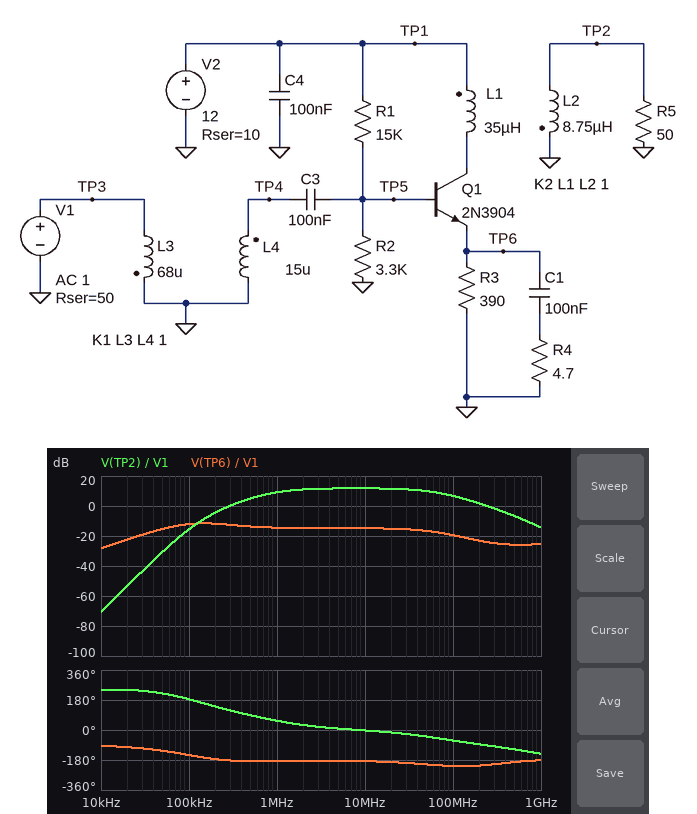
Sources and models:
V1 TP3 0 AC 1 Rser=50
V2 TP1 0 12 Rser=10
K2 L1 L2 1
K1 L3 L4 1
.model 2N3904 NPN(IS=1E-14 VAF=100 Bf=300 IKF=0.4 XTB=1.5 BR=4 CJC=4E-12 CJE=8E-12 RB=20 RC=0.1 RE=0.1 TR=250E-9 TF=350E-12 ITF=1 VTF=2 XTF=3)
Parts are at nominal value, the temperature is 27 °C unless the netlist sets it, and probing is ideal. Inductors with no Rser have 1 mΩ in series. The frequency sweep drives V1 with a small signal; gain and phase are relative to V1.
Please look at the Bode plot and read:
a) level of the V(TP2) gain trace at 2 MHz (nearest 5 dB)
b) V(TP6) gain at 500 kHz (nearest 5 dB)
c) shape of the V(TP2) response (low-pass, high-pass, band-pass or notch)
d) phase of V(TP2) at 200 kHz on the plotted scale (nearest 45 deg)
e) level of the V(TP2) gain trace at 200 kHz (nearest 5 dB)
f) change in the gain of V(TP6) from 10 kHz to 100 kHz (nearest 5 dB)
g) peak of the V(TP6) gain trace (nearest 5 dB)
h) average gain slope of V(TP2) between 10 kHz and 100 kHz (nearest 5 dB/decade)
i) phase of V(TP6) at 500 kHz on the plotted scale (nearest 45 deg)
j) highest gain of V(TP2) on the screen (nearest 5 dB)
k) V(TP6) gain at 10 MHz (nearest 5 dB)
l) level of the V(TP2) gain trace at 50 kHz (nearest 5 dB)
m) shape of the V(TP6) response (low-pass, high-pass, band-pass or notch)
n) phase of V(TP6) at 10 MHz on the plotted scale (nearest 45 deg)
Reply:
10 dB
-15 dB
band-pass
135 deg
-5 dB
15 dB
-10 dB
55 dB/decade
-180 deg
10 dB
-15 dB
-30 dB
band-pass
-180 deg
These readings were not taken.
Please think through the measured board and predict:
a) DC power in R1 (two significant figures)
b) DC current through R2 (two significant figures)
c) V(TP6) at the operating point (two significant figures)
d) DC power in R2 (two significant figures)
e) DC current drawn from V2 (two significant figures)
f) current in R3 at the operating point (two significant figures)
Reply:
6.4 mW
640 µA
1.4 V
1.4 mW
4.3 mA
3.7 mA
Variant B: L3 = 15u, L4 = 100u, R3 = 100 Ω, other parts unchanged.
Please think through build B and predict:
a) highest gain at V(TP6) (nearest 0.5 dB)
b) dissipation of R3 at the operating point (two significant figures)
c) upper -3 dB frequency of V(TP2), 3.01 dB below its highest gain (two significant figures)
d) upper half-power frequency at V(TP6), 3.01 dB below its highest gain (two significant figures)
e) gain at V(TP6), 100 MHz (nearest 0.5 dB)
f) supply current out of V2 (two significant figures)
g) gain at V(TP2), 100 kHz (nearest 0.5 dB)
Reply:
3.5 dB
17 mW
6.2 MHz
5.3 MHz
-22.5 dB
14 mA
-10.0 dB
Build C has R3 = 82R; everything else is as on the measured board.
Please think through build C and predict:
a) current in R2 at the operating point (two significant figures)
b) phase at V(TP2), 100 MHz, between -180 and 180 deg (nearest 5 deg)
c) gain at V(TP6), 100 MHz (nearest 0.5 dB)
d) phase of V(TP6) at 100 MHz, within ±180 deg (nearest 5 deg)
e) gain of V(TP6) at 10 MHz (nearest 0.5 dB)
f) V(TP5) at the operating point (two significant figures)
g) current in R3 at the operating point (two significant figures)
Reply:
610 µA
-75 deg
-18.0 dB
130 deg
-10.0 dB
2.0 V
16 mA
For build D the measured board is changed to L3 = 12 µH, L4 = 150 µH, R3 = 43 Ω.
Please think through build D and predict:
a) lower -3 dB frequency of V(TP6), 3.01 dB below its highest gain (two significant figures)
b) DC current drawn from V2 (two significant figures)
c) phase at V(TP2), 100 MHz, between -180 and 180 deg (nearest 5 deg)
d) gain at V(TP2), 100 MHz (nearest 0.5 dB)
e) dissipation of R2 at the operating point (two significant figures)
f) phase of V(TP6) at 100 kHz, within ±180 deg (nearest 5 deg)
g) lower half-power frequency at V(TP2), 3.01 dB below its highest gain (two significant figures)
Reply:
370 kHz
27 mA
-95 deg
1.5 dB
1.1 mW
-105 deg
830 kHz
